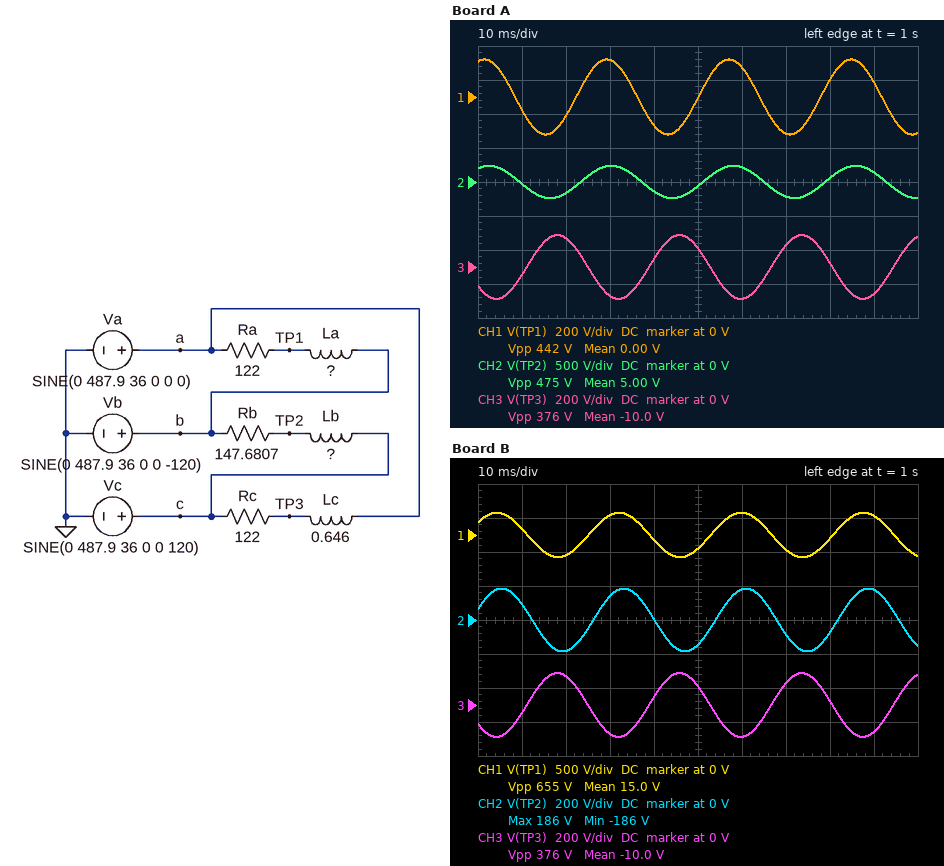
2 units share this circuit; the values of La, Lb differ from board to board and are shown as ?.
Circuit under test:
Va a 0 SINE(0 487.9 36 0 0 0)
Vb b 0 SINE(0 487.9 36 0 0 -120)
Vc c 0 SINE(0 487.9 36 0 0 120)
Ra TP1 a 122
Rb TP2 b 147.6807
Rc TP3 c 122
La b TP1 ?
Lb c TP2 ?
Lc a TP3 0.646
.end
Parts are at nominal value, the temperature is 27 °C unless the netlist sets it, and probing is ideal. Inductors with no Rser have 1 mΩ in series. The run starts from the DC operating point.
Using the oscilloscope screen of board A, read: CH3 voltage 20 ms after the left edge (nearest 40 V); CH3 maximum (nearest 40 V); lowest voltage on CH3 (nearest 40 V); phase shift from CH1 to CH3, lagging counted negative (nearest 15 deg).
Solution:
160 V
200 V
-200 V
150 deg
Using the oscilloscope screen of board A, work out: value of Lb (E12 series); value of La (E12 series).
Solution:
390 mH
820 mH
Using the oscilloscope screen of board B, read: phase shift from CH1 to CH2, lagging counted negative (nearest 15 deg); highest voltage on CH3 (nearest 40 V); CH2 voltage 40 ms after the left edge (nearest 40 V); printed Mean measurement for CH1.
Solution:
-15 deg
200 V
0 V
15.0 V
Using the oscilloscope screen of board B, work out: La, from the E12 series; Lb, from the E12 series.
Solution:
1.5 H
560 mH
